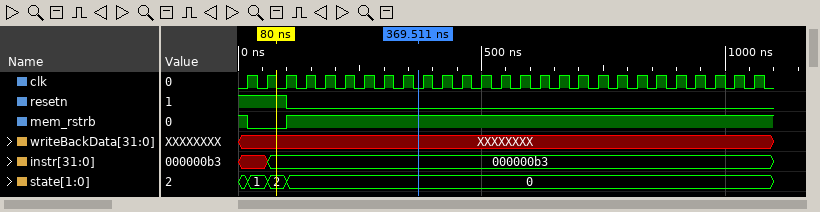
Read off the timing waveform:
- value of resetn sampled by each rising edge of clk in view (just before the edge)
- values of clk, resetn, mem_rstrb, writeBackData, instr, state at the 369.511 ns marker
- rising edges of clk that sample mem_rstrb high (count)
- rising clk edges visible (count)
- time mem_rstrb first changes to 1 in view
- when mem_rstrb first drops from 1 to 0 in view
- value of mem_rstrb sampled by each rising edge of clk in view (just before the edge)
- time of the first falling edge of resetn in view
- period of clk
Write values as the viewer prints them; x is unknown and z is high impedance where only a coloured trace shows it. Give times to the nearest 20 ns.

1 1 1 0 0 0 0 0 0 0 0 0 0 0 0 0 0 0 0 0 0 0 0 0 0 0 0
clk=0, resetn=0, mem_rstrb=1, writeBackData=XXXXXXXX, instr=000000b3, state=0
25
27
100 ns
20 ns
1 0 0 1 1 1 1 1 1 1 1 1 1 1 1 1 1 1 1 1 1 1 1 1 1 1 1
100 ns
40 ns
